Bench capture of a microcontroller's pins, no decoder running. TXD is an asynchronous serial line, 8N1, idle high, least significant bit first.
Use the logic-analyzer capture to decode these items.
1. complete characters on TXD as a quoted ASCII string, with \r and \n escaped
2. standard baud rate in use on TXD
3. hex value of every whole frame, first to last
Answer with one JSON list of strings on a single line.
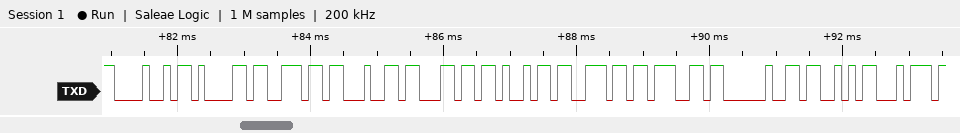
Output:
["\"Handling St\"", "9600 baud", "48 61 6E 64 6C 69 6E 67 20 53 74"]
